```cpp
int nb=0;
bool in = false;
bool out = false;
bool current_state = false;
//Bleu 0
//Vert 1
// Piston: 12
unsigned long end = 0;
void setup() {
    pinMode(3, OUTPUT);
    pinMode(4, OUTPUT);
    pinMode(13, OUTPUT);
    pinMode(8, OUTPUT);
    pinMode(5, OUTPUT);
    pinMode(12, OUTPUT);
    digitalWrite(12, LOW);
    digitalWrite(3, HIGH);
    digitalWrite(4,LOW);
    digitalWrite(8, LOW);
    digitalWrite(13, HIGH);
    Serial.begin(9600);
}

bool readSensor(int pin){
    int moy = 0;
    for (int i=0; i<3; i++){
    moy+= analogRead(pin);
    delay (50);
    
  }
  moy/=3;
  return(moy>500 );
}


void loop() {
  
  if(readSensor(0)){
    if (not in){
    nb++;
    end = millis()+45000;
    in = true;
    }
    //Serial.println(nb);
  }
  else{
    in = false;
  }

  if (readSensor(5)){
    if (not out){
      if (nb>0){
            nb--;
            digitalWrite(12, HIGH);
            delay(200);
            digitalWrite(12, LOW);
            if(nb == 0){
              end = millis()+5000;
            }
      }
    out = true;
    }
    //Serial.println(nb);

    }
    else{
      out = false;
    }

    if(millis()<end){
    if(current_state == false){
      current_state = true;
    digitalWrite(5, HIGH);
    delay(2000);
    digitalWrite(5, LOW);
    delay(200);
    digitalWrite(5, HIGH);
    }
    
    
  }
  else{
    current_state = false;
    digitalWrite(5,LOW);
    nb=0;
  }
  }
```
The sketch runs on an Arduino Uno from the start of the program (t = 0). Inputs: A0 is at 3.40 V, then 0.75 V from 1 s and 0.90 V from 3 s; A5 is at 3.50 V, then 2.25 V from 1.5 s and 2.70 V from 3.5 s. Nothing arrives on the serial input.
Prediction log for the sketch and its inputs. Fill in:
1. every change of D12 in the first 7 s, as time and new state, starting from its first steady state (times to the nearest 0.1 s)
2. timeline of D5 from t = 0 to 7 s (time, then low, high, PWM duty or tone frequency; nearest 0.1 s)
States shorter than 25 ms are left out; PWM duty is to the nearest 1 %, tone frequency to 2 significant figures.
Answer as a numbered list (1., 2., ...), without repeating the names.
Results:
1. 0 s low; 0.3 s high; 0.5 s low
2. 0 s low; 0.5 s high; 2.5 s low; 2.7 s high; 5.7 s low
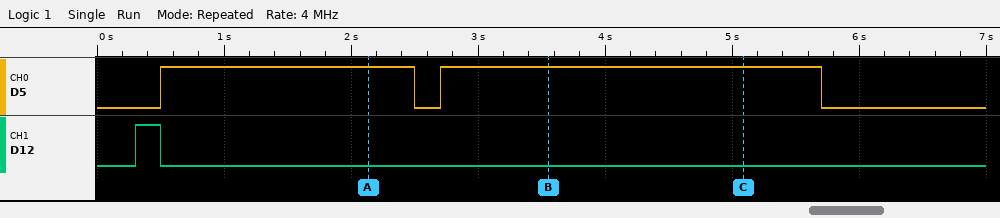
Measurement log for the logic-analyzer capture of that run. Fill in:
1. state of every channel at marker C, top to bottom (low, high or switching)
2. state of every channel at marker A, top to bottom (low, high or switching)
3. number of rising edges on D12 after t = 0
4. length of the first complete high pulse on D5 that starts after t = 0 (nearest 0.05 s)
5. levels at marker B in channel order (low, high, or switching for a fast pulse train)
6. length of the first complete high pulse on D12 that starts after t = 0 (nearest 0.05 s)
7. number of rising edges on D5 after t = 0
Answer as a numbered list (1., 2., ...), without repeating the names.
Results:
1. D5 high, D12 low
2. D5 high, D12 low
3. 1
4. 2.00 s
5. D5 high, D12 low
6. 0.20 s
7. 2
